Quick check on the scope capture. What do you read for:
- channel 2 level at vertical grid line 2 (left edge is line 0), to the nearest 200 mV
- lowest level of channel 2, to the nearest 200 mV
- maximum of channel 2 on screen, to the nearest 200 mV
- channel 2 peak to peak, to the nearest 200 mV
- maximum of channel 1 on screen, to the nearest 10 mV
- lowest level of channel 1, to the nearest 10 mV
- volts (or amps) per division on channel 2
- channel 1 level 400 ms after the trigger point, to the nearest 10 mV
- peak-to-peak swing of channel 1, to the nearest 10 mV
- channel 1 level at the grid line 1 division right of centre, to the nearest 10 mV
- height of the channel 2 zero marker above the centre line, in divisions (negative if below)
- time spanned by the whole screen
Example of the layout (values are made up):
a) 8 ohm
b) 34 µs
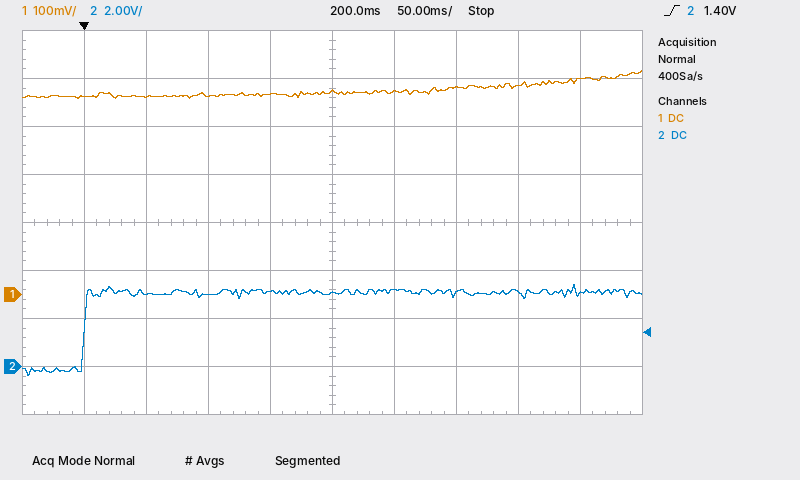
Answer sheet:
a) 3.0 V
b) -400 mV
c) 3.4 V
d) 3.8 V
e) 470 mV
f) 410 mV
g) 2 V
h) 450 mV
i) 60 mV
j) 420 mV
k) -3.0 div
l) 500 ms
